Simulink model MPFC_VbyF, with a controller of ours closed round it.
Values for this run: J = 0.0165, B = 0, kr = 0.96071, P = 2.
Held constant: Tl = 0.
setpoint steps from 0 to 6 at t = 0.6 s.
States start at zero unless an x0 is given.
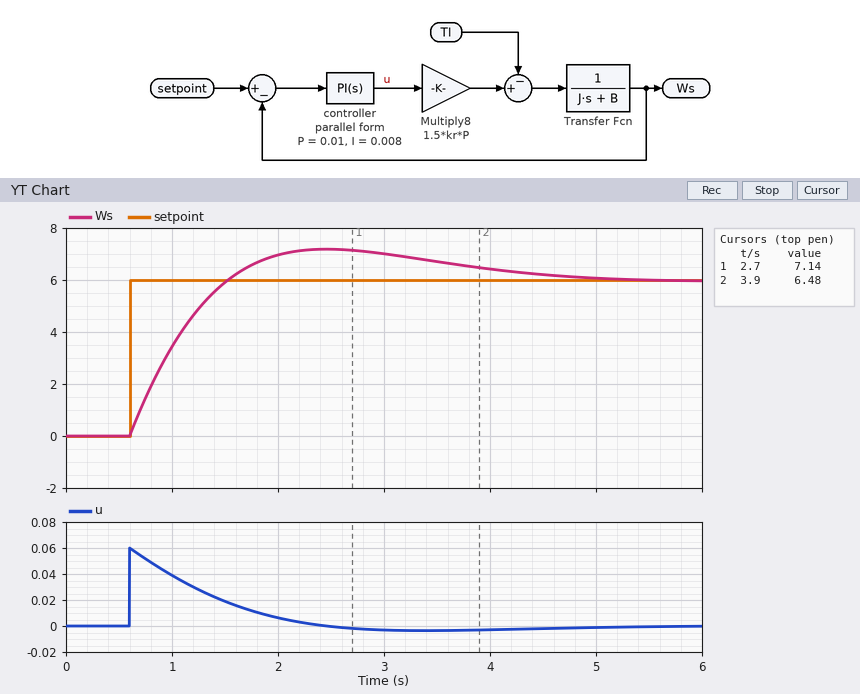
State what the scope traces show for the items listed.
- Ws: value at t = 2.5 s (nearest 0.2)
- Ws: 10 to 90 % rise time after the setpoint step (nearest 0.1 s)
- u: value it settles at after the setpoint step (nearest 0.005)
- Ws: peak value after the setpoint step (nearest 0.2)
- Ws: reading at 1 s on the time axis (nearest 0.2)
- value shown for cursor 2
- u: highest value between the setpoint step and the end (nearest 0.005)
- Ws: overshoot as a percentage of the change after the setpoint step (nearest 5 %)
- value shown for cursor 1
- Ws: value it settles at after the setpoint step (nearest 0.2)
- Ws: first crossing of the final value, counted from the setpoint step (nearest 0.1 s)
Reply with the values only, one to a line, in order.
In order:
7.2
0.7 s
0.000
7.2
3.4
6.48
0.060
20 %
7.14
6.0
0.9 s
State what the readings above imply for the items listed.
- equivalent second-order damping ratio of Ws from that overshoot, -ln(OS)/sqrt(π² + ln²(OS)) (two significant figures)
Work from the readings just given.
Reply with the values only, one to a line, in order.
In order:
0.46
